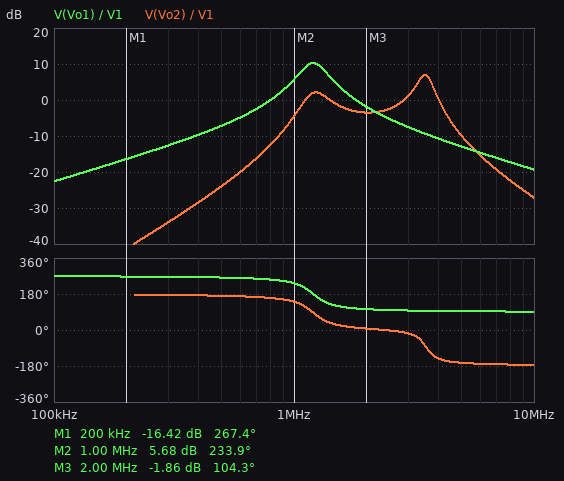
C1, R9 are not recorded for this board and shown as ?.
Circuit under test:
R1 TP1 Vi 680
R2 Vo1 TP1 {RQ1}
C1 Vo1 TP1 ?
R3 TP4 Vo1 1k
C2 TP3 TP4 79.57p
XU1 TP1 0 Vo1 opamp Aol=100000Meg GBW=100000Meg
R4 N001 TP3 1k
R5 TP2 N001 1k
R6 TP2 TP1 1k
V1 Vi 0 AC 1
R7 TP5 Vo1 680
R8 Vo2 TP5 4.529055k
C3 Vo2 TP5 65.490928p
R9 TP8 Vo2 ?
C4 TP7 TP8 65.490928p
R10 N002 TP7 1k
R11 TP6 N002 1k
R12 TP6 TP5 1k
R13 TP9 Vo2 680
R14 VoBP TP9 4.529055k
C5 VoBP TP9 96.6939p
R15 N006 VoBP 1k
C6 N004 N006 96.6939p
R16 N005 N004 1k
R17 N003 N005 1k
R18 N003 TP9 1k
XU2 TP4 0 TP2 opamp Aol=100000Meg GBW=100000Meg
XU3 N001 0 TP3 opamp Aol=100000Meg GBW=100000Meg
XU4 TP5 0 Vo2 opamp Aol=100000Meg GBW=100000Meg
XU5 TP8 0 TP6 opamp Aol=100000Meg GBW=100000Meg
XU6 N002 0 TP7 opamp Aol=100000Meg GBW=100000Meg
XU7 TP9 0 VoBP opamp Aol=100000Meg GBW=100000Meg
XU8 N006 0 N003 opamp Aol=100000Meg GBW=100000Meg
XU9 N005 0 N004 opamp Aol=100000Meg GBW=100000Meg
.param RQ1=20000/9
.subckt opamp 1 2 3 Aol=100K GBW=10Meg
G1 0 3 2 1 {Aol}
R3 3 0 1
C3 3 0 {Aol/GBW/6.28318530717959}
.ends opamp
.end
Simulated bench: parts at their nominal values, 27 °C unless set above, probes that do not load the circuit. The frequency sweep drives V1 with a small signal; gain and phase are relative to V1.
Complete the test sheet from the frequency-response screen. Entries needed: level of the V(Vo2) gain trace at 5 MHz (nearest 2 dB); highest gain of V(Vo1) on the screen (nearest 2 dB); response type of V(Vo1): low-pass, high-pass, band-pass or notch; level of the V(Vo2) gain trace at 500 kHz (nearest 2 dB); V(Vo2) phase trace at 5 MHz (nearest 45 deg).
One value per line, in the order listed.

-10 dB
10 dB
band-pass
-24 dB
-180 deg
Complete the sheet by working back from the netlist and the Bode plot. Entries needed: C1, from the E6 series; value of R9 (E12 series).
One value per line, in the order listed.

220 pF
470 Ω
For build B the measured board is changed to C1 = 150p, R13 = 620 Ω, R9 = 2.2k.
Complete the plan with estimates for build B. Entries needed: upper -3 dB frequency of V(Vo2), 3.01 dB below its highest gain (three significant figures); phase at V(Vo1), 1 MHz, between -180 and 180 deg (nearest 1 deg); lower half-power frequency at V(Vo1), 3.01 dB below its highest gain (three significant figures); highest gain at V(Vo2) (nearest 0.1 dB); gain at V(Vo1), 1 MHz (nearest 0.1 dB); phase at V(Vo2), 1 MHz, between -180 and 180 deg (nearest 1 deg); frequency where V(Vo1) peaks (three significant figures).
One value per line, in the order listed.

1.74 MHz
-113 deg
1.24 MHz
25.7 dB
2.1 dB
139 deg
1.46 MHz
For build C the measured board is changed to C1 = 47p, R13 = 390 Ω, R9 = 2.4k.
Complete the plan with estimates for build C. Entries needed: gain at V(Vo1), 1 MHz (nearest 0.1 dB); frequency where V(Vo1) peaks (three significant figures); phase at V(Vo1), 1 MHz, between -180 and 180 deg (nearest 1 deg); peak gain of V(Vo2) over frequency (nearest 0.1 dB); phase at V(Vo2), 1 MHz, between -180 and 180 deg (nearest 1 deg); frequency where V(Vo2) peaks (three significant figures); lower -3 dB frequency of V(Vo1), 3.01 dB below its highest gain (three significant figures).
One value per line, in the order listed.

-1.6 dB
2.60 MHz
-105 deg
20.8 dB
145 deg
1.66 MHz
1.95 MHz
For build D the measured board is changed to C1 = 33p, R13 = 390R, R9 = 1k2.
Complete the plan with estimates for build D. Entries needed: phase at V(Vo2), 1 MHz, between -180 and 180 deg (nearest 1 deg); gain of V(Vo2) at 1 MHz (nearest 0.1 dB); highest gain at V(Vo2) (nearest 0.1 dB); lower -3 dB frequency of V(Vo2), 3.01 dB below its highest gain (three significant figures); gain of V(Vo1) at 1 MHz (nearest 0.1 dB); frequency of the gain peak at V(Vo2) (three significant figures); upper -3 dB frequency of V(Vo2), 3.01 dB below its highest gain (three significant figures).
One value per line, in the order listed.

158 deg
-2.9 dB
24.0 dB
2.04 MHz
-2.0 dB
2.27 MHz
2.64 MHz
